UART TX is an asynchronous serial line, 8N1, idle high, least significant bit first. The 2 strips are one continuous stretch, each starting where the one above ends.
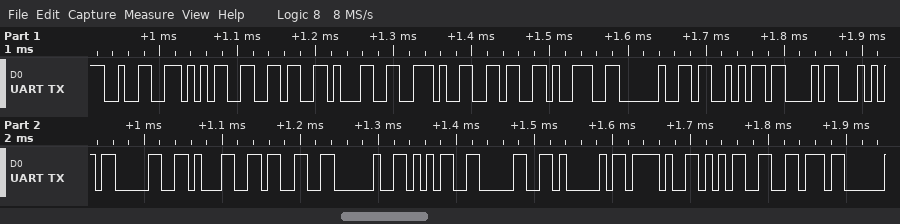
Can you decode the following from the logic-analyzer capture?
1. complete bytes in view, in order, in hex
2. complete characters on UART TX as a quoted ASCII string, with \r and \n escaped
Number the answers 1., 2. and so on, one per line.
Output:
1. 32 35 36 31 2E 36 39 20 53 43 54 30 31 33 20 35 30 41 2F 35 76
2. "2561.69 SCT013 50A/5v"
